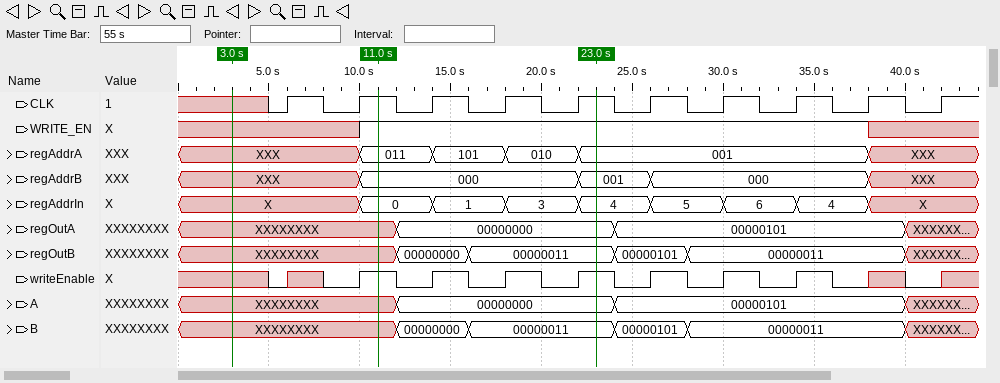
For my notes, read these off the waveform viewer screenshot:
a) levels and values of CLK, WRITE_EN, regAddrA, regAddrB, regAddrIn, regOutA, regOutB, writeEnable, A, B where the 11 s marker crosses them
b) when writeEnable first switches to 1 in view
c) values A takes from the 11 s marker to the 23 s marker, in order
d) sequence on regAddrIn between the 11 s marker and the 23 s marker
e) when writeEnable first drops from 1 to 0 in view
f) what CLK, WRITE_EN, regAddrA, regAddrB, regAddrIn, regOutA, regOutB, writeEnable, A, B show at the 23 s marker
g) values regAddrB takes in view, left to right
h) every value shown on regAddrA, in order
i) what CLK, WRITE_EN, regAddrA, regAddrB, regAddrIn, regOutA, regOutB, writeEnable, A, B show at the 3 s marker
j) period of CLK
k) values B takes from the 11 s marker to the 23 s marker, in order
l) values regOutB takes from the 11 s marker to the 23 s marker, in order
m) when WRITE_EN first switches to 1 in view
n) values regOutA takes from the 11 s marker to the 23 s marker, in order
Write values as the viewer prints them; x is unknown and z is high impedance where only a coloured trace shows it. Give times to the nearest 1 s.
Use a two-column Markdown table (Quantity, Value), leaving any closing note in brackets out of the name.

| Quantity | Value |
|---|---|
| levels and values of CLK, WRITE_EN, regAddrA, regAddrB, regAddrIn, regOutA, regOutB, writeEnable, A, B where the 11 s marker crosses them | CLK=1, WRITE_EN=1, regAddrA=011, regAddrB=000, regAddrIn=0, regOutA=XXXXXXXX, regOutB=XXXXXXXX, writeEnable=1, A=XXXXXXXX, B=XXXXXXXX |
| when writeEnable first switches to 1 in view | 10 s |
| values A takes from the 11 s marker to the 23 s marker, in order | XXXXXXXX, 00000000 |
| sequence on regAddrIn between the 11 s marker and the 23 s marker | 0, 1, 3, 4 |
| when writeEnable first drops from 1 to 0 in view | 12 s |
| what CLK, WRITE_EN, regAddrA, regAddrB, regAddrIn, regOutA, regOutB, writeEnable, A, B show at the 23 s marker | CLK=1, WRITE_EN=1, regAddrA=001, regAddrB=001, regAddrIn=4, regOutA=00000000, regOutB=00000011, writeEnable=1, A=00000000, B=00000011 |
| values regAddrB takes in view, left to right | XXX, 000, 001, 000, XXX |
| every value shown on regAddrA, in order | XXX, 011, 101, 010, 001, XXX |
| what CLK, WRITE_EN, regAddrA, regAddrB, regAddrIn, regOutA, regOutB, writeEnable, A, B show at the 3 s marker | CLK=x, WRITE_EN=x, regAddrA=XXX, regAddrB=XXX, regAddrIn=X, regOutA=XXXXXXXX, regOutB=XXXXXXXX, writeEnable=x, A=XXXXXXXX, B=XXXXXXXX |
| period of CLK | 4 s |
| values B takes from the 11 s marker to the 23 s marker, in order | XXXXXXXX, 00000000, 00000011 |
| values regOutB takes from the 11 s marker to the 23 s marker, in order | XXXXXXXX, 00000000, 00000011 |
| when WRITE_EN first switches to 1 in view | 10 s |
| values regOutA takes from the 11 s marker to the 23 s marker, in order | XXXXXXXX, 00000000 |
